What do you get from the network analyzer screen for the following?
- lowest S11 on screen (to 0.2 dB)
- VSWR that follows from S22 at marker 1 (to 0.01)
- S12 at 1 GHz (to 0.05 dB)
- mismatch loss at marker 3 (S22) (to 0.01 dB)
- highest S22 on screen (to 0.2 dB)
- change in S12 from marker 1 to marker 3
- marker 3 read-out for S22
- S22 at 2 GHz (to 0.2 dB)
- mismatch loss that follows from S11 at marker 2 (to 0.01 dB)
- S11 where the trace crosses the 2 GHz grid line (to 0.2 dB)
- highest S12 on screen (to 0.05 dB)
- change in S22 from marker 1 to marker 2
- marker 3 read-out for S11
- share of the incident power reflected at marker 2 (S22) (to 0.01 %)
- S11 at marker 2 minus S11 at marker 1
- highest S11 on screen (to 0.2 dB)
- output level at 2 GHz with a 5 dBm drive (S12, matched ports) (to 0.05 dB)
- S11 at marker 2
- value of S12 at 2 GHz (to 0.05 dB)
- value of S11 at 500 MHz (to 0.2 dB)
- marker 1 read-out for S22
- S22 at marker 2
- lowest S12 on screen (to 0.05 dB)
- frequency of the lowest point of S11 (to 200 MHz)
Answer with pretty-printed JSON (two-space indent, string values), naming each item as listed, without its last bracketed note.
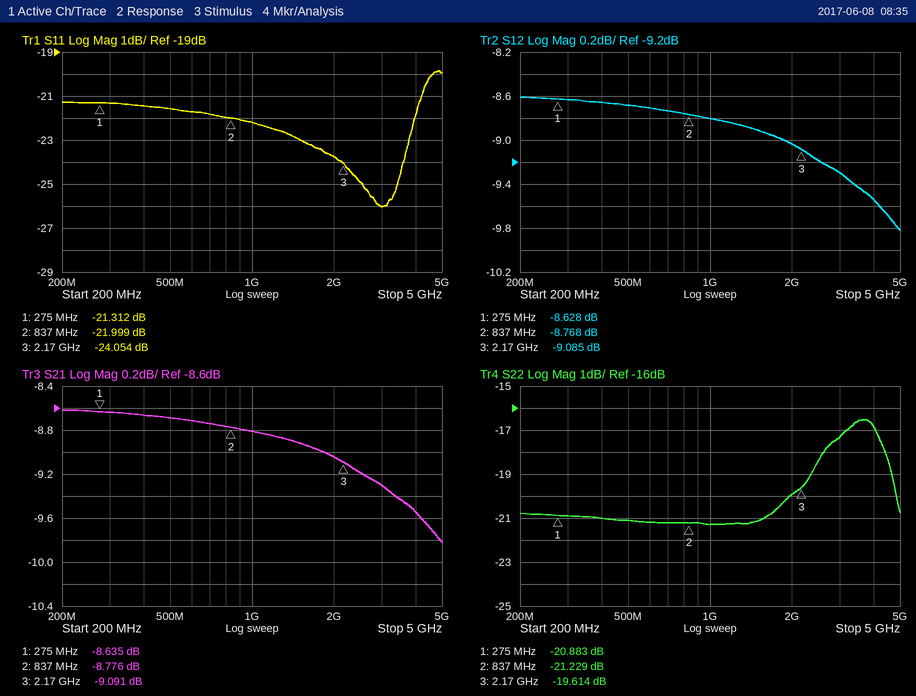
{
  "lowest S11 on screen": "-26.0 dB",
  "VSWR that follows from S22 at marker 1": "1.20",
  "S12 at 1 GHz": "-8.80 dB",
  "mismatch loss at marker 3 (S22)": "0.05 dB",
  "highest S22 on screen": "-16.6 dB",
  "change in S12 from marker 1 to marker 3": "-0.457 dB",
  "marker 3 read-out for S22": "-19.614 dB",
  "S22 at 2 GHz": "-20.0 dB",
  "mismatch loss that follows from S11 at marker 2": "0.03 dB",
  "S11 where the trace crosses the 2 GHz grid line": "-23.8 dB",
  "highest S12 on screen": "-8.60 dB",
  "change in S22 from marker 1 to marker 2": "-0.346 dB",
  "marker 3 read-out for S11": "-24.054 dB",
  "share of the incident power reflected at marker 2 (S22)": "0.75 %",
  "S11 at marker 2 minus S11 at marker 1": "-0.687 dB",
  "highest S11 on screen": "-19.8 dB",
  "output level at 2 GHz with a 5 dBm drive (S12, matched ports)": "-4.05 dBm",
  "S11 at marker 2": "-21.999 dB",
  "value of S12 at 2 GHz": "-9.05 dB",
  "value of S11 at 500 MHz": "-21.6 dB",
  "marker 1 read-out for S22": "-20.883 dB",
  "S22 at marker 2": "-21.229 dB",
  "lowest S12 on screen": "-9.80 dB",
  "frequency of the lowest point of S11": "3.0 GHz"
}
